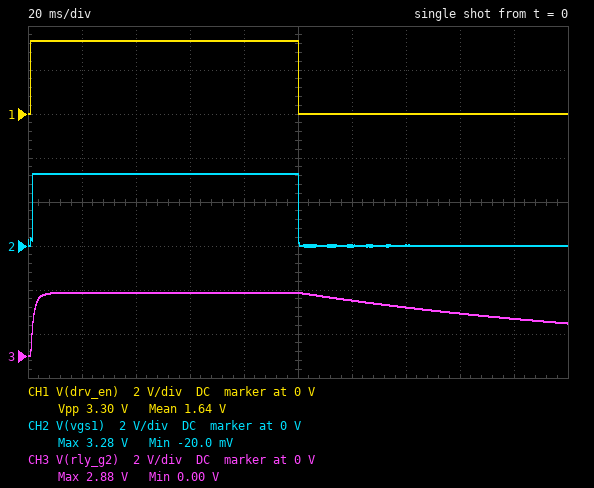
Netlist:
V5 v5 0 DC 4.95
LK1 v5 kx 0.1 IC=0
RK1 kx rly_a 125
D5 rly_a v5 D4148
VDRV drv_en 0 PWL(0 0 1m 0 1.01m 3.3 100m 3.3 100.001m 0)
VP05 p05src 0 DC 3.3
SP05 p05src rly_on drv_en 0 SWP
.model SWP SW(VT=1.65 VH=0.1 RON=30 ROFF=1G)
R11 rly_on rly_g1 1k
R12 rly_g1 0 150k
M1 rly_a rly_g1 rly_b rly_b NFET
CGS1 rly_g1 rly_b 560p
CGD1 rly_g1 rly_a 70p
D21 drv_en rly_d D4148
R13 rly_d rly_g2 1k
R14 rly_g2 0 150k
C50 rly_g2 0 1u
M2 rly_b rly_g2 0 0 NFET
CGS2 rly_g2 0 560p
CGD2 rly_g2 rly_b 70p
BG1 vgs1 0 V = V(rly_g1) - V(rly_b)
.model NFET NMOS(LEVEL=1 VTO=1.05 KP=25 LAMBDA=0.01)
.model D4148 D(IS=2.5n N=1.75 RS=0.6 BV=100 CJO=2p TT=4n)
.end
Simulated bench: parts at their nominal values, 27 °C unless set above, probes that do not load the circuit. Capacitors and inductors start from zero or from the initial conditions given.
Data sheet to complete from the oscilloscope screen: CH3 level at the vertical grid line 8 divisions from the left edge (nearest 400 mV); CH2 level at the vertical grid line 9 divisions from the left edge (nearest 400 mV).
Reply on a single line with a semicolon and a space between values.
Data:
2.0 V; 0 V
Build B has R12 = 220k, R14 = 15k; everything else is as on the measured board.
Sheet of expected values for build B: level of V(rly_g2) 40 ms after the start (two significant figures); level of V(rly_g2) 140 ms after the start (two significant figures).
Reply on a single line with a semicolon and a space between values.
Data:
2.6 V; 180 mV
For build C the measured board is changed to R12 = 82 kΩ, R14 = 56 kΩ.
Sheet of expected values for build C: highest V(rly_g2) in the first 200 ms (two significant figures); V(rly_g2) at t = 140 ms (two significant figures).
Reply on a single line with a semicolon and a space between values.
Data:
2.8 V; 1.4 V
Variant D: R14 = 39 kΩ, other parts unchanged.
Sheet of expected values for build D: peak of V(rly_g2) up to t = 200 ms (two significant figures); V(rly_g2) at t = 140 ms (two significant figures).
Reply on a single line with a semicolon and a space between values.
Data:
2.8 V; 990 mV
